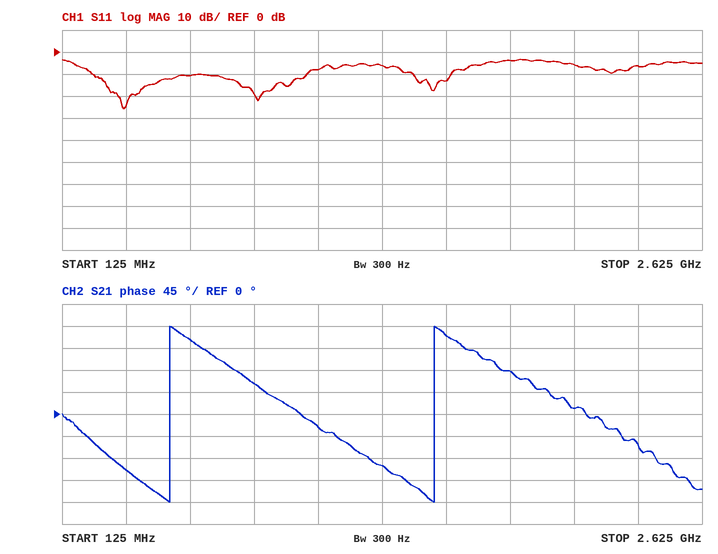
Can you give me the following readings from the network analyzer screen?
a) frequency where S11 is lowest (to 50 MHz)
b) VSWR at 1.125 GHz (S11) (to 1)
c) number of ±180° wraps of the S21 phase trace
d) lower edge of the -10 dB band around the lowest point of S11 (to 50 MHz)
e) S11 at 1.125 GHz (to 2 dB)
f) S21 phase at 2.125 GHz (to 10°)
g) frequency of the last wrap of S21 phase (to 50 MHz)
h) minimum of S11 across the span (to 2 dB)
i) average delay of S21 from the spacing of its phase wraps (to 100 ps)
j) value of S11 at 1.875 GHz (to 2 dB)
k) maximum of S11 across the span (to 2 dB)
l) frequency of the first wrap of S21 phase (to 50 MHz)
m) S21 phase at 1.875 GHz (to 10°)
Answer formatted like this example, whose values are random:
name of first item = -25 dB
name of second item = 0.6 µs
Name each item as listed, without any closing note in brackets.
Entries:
frequency where S11 is lowest = 350 MHz
VSWR at 1.125 GHz (S11) = 2
number of ±180° wraps of the S21 phase trace = 2
lower edge of the -10 dB band around the lowest point of S11 = 250 MHz
S11 at 1.125 GHz = -8 dB
S21 phase at 2.125 GHz = 10°
frequency of the last wrap of S21 phase = 1.60 GHz
minimum of S11 across the span = -26 dB
average delay of S21 from the spacing of its phase wraps = 1.0 ns
value of S11 at 1.875 GHz = -4 dB
maximum of S11 across the span = -4 dB
frequency of the first wrap of S21 phase = 550 MHz
S21 phase at 1.875 GHz = 90°
